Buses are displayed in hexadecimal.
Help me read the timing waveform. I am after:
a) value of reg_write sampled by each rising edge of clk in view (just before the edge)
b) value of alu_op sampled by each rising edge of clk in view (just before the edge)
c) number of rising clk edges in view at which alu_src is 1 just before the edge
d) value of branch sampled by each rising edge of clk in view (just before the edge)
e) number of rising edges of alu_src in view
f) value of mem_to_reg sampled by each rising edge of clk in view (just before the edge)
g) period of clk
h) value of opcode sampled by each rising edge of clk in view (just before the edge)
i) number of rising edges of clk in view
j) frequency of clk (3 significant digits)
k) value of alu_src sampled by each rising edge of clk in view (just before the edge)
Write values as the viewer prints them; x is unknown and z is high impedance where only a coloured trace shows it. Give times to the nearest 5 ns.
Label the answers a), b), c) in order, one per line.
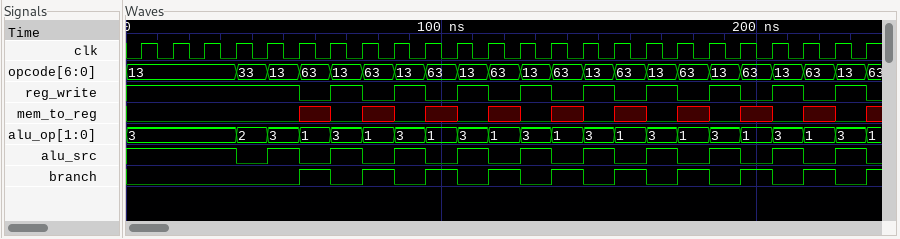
a) 1 1 1 1 1 1 0 1 0 1 0 1 0 1 0 1 0 1 0 1 0 1 0 1
b) 3, 3, 3, 3, 2, 3, 1, 3, 1, 3, 1, 3, 1, 3, 1, 3, 1, 3, 1, 3, 1, 3, 1, 3
c) 14
d) 0 0 0 0 0 0 1 0 1 0 1 0 1 0 1 0 1 0 1 0 1 0 1 0
e) 10
f) 0 0 0 0 0 0 x 0 x 0 x 0 x 0 x 0 x 0 x 0 x 0 x 0
g) 10 ns
h) 13, 13, 13, 13, 33, 13, 63, 13, 63, 13, 63, 13, 63, 13, 63, 13, 63, 13, 63, 13, 63, 13, 63, 13
i) 24
j) 100 MHz
k) 1 1 1 1 0 1 0 1 0 1 0 1 0 1 0 1 0 1 0 1 0 1 0 1
